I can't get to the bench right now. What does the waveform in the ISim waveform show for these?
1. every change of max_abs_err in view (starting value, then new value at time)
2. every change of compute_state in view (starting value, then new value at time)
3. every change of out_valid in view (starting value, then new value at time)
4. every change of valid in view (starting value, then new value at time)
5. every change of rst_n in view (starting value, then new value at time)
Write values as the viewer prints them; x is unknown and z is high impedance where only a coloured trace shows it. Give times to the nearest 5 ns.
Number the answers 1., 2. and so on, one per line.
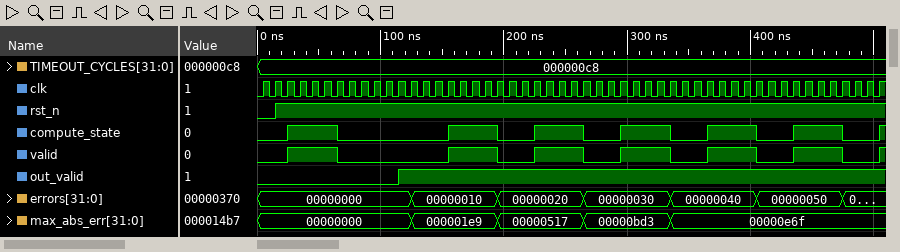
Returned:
1. 00000000, 000001e9 at 125 ns, 00000517 at 195 ns, 00000bd3 at 265 ns, 00000e6f at 335 ns
2. 0, 1 at 25 ns, 0 at 65 ns, 1 at 155 ns, 0 at 195 ns, 1 at 225 ns, 0 at 265 ns, 1 at 295 ns, 0 at 335 ns, 1 at 365 ns, 0 at 405 ns, 1 at 435 ns, 0 at 475 ns, 1 at 505 ns
3. 0, 1 at 115 ns
4. 0, 1 at 25 ns, 0 at 65 ns, 1 at 155 ns, 0 at 195 ns, 1 at 225 ns, 0 at 265 ns, 1 at 295 ns, 0 at 335 ns, 1 at 365 ns, 0 at 405 ns, 1 at 435 ns, 0 at 475 ns, 1 at 505 ns
5. 0, 1 at 15 ns
